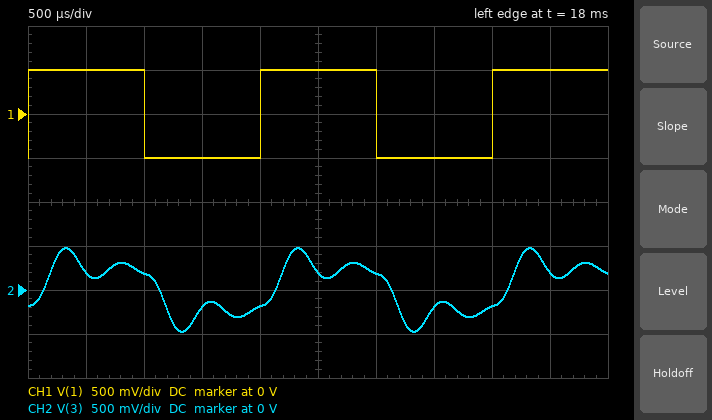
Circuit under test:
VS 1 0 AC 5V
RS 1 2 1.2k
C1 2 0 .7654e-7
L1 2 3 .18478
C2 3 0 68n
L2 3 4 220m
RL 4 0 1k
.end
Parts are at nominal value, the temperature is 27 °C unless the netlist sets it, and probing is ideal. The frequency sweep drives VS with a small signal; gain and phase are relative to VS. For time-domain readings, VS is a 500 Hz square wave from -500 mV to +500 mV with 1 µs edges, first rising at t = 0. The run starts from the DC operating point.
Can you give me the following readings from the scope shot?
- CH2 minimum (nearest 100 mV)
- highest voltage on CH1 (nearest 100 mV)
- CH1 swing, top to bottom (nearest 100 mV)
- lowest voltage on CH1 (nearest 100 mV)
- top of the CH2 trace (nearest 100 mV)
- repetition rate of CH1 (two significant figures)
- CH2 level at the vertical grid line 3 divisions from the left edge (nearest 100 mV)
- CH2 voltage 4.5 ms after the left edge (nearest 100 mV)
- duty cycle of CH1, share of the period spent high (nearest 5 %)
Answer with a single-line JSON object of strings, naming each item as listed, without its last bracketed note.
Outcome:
{"CH2 minimum": "-500 mV", "highest voltage on CH1": "500 mV", "CH1 swing, top to bottom": "1.0 V", "lowest voltage on CH1": "-500 mV", "top of the CH2 trace": "500 mV", "repetition rate of CH1": "500 Hz", "CH2 level at the vertical grid line 3 divisions from the left edge": "-200 mV", "CH2 voltage 4.5 ms after the left edge": "200 mV", "duty cycle of CH1, share of the period spent high": "50 %"}
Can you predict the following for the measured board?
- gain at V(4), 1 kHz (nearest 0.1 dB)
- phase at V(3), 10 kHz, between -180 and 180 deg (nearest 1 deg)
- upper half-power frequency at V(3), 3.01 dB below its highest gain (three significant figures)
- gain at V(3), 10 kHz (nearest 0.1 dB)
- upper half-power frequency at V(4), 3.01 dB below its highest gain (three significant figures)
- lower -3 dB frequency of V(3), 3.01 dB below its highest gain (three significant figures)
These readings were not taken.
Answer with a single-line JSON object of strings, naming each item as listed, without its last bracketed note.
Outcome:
{"gain at V(4), 1 kHz": "-8.5 dB", "phase at V(3), 10 kHz, between -180 and 180 deg": "100 deg", "upper half-power frequency at V(3), 3.01 dB below its highest gain": "2.29 kHz", "gain at V(3), 10 kHz": "-48.8 dB", "upper half-power frequency at V(4), 3.01 dB below its highest gain": "2.25 kHz", "lower -3 dB frequency of V(3), 3.01 dB below its highest gain": "1.67 kHz"}
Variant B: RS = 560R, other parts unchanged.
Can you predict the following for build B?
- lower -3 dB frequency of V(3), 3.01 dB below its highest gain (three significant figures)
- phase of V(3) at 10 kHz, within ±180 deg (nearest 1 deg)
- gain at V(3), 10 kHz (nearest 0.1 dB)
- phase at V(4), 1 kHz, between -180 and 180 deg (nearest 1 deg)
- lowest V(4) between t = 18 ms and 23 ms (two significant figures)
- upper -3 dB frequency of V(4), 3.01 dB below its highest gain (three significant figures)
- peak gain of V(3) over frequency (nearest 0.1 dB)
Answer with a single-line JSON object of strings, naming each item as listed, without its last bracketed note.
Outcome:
{"lower -3 dB frequency of V(3), 3.01 dB below its highest gain": "1.63 kHz", "phase of V(3) at 10 kHz, within ±180 deg": "111 deg", "gain at V(3), 10 kHz": "-42.6 dB", "phase at V(4), 1 kHz, between -180 and 180 deg": "-84 deg", "lowest V(4) between t = 18 ms and 23 ms": "-340 mV", "upper -3 dB frequency of V(4), 3.01 dB below its highest gain": "2.14 kHz", "peak gain of V(3) over frequency": "5.5 dB"}
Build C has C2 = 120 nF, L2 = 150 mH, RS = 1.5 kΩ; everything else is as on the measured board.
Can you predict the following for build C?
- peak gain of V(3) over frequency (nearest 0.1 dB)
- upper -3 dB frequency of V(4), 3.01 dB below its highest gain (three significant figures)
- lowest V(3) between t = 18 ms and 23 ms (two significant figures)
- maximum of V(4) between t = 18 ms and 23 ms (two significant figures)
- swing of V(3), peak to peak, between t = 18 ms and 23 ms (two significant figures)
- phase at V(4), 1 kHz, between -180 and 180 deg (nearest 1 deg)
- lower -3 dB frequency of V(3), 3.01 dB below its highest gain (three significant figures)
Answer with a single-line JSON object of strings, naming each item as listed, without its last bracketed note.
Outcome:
{"peak gain of V(3) over frequency": "-2.6 dB", "upper -3 dB frequency of V(4), 3.01 dB below its highest gain": "1.92 kHz", "lowest V(3) between t = 18 ms and 23 ms": "-370 mV", "maximum of V(4) between t = 18 ms and 23 ms": "260 mV", "swing of V(3), peak to peak, between t = 18 ms and 23 ms": "740 mV", "phase at V(4), 1 kHz, between -180 and 180 deg": "-98 deg", "lower -3 dB frequency of V(3), 3.01 dB below its highest gain": "890 Hz"}
